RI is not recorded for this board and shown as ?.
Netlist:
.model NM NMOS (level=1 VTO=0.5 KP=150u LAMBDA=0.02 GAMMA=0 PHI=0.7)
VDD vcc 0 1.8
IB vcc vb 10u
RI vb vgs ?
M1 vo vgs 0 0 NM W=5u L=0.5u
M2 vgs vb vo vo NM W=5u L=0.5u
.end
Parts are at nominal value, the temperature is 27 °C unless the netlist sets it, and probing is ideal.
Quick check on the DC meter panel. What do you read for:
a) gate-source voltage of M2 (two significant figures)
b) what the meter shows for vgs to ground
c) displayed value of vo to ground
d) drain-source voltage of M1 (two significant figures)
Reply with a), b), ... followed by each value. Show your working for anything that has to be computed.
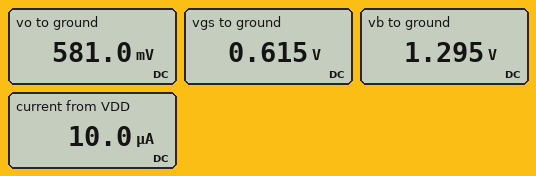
a) 1.295 V - 581 mV = 710 mV
b) 0.615 V
c) 581.0 mV
d) 581 mV = 580 mV
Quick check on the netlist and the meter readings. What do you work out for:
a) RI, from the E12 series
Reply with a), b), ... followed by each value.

a) 68 kΩ
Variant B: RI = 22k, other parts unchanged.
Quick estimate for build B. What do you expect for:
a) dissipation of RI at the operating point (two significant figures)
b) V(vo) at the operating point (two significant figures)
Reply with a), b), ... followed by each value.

a) 2.2 µW
b) 220 mV
